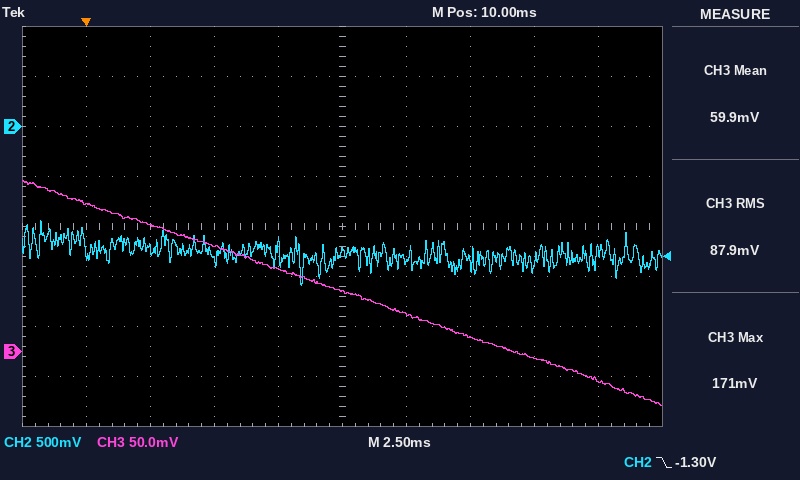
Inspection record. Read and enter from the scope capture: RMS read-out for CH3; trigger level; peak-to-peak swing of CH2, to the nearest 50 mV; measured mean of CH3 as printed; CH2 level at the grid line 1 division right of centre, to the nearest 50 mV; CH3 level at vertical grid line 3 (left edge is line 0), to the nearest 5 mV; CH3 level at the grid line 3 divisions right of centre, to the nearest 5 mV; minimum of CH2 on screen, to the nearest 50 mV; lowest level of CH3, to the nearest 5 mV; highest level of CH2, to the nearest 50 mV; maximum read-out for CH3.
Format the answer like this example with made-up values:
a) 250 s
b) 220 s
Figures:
a) 87.9 mV
b) -1.30 V
c) 650 mV
d) 59.9 mV
e) -1.35 V
f) 105 mV
g) -5 mV
h) -1.60 V
i) -55 mV
j) -950 mV
k) 171 mV
